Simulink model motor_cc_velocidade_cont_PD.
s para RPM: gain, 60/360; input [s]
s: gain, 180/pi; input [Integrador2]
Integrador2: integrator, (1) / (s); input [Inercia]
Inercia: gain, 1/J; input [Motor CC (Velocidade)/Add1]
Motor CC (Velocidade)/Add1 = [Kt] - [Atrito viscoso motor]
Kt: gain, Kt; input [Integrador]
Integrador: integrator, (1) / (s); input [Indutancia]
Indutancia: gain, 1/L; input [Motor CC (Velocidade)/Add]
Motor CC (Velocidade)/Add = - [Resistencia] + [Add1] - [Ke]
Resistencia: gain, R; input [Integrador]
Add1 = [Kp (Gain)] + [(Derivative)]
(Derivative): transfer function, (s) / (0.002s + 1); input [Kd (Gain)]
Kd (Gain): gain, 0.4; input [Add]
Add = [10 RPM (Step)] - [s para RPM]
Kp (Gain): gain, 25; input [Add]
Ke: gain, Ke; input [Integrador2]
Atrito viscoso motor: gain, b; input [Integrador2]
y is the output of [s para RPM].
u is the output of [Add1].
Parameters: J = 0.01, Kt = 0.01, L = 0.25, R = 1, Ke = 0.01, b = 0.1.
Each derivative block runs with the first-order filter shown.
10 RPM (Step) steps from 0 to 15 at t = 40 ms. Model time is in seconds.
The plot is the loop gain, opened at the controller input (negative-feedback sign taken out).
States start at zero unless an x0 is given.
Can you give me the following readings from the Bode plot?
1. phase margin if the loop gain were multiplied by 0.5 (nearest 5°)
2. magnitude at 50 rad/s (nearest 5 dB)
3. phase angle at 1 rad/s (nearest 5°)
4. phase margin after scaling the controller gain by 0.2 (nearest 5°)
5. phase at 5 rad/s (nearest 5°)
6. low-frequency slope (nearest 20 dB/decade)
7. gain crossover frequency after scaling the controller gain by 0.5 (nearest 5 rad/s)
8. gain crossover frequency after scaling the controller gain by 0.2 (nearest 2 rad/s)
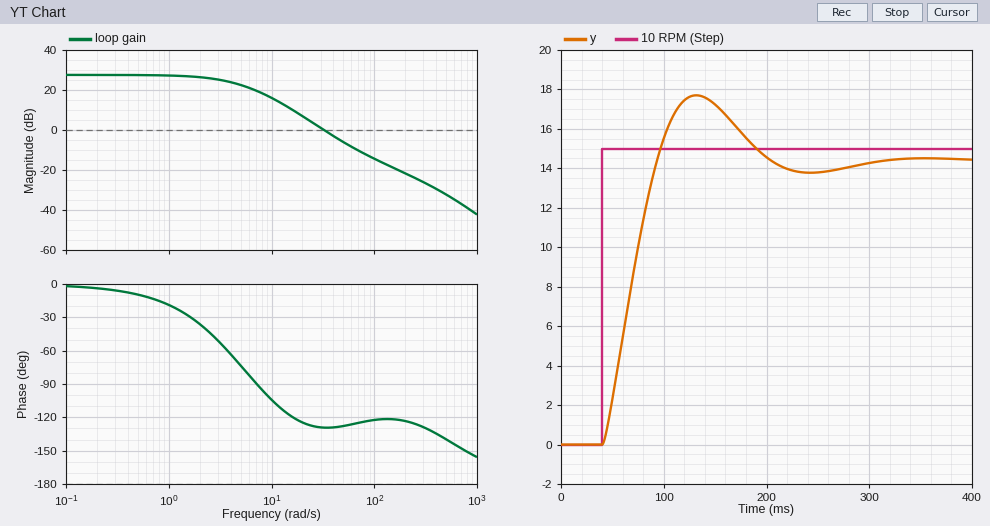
55°
-5 dB
-20°
70°
-75°
0 dB/decade
20 rad/s
12 rad/s
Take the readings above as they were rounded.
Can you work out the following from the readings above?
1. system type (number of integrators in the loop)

0
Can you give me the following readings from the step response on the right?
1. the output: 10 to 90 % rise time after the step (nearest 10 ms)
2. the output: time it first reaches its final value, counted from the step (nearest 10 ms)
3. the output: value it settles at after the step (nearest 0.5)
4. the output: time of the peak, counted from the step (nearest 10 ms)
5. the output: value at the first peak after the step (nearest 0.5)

40 ms
50 ms
14.5
90 ms
17.5
